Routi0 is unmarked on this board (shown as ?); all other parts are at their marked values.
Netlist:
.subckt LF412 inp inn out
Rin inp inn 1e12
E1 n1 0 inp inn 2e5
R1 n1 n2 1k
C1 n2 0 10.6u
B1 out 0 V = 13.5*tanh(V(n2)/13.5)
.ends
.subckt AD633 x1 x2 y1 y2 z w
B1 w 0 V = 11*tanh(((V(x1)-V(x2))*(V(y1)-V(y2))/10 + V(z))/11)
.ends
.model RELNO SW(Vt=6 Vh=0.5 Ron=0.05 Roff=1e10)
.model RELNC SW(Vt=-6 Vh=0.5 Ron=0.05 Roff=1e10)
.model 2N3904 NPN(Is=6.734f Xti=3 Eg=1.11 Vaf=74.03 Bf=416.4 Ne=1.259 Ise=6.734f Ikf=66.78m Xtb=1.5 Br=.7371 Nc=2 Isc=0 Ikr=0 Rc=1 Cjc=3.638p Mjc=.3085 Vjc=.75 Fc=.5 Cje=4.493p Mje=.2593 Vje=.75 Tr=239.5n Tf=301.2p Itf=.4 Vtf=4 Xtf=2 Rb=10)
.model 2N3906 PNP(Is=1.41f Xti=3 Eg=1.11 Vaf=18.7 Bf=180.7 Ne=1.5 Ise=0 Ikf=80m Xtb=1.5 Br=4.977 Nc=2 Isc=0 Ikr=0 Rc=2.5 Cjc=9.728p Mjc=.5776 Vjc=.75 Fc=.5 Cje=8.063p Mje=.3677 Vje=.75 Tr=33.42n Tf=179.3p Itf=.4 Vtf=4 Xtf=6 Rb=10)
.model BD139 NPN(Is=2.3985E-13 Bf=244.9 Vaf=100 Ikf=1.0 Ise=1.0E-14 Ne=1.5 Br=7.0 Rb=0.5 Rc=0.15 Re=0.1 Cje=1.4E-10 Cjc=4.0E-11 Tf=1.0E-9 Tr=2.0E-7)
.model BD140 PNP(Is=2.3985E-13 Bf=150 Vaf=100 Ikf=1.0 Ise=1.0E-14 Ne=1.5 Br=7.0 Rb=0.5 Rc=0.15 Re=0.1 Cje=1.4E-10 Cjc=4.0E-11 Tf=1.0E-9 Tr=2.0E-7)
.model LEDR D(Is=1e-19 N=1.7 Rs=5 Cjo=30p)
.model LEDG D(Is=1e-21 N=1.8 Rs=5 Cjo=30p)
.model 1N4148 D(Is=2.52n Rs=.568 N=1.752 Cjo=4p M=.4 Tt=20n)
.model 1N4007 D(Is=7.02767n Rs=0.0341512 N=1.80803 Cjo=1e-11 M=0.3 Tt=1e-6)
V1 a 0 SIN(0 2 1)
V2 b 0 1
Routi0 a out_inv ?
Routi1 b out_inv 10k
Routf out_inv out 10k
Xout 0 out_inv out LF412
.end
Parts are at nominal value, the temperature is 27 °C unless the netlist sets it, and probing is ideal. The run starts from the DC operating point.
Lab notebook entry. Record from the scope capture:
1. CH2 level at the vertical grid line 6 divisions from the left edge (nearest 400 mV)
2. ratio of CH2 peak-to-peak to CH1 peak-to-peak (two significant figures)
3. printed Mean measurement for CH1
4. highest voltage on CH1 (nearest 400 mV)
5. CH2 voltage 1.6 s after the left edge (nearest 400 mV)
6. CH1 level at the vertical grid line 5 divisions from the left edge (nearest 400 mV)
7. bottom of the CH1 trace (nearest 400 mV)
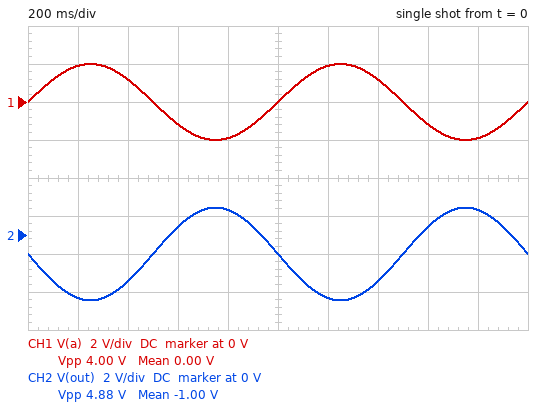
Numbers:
-3.2 V
1.2
0.00 V
2.0 V
400 mV
0 V
-2.0 V
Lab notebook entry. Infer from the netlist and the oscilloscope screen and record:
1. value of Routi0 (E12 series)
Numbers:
8.2 kΩ
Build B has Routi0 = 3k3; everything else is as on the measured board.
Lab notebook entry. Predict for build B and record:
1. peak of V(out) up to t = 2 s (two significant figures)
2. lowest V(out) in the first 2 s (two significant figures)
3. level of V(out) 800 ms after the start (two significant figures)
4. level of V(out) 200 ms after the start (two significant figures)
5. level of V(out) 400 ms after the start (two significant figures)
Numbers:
5.1 V
-7.1 V
4.8 V
-6.8 V
-4.6 V
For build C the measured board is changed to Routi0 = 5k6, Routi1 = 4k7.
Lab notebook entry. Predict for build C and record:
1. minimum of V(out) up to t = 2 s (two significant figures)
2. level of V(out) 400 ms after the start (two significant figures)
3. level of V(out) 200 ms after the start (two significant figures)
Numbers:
-5.7 V
-4.2 V
-5.5 V
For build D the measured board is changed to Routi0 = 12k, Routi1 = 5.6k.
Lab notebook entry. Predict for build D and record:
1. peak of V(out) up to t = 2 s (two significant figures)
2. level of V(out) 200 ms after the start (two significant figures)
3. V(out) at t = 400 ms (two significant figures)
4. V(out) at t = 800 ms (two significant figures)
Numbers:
-120 mV
-3.4 V
-2.8 V
-200 mV
